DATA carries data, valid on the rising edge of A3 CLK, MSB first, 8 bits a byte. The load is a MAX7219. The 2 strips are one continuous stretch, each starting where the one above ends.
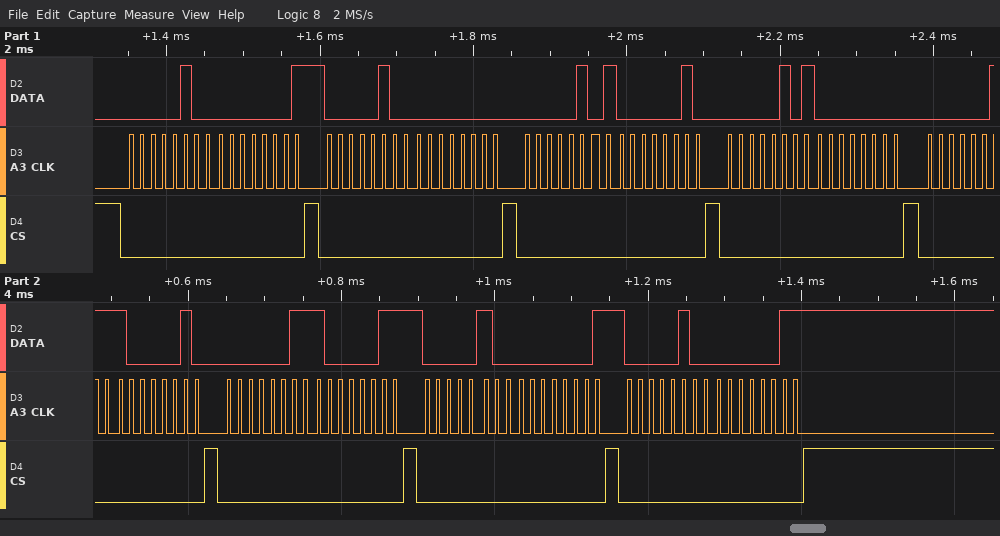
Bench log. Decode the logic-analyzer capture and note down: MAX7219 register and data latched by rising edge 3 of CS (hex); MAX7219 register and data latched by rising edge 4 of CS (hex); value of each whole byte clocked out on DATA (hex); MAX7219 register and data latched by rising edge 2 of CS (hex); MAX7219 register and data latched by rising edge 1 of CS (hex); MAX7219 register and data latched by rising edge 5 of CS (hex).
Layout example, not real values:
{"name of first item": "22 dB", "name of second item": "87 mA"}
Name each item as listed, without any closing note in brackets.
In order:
{"MAX7219 register and data latched by rising edge 3 of CS": "register 0x5, data 0x02", "MAX7219 register and data latched by rising edge 4 of CS": "register 0x5, data 0x00", "value of each whole byte clocked out on DATA": "0x04 0x01 0x04 0x00 0x05 0x02 0x05 0x00 0x03 0x82 0x03 0x83 0x04 0x01 0x04 0x03", "MAX7219 register and data latched by rising edge 2 of CS": "register 0x4, data 0x00", "MAX7219 register and data latched by rising edge 1 of CS": "register 0x4, data 0x01", "MAX7219 register and data latched by rising edge 5 of CS": "register 0x3, data 0x82"}
